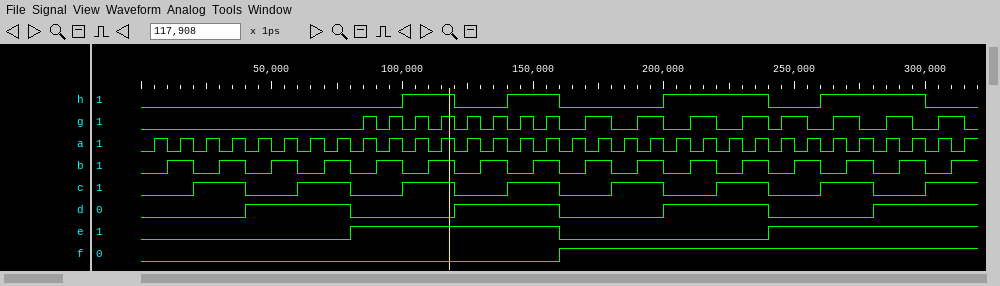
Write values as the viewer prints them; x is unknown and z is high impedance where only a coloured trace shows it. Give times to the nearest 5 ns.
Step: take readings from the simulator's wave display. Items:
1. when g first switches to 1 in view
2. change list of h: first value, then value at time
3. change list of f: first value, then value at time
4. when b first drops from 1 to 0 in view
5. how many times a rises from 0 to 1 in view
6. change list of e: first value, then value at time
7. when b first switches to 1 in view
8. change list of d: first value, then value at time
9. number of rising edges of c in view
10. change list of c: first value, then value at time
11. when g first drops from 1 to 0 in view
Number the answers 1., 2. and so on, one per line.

1. 85 ns
2. 0, 1 at 100 ns, 0 at 120 ns, 1 at 140 ns, 0 at 160 ns, 1 at 200 ns, 0 at 240 ns, 1 at 260 ns, 0 at 300 ns
3. 0, 1 at 160 ns
4. 20 ns
5. 32
6. 0, 1 at 80 ns, 0 at 160 ns, 1 at 240 ns
7. 10 ns
8. 0, 1 at 40 ns, 0 at 80 ns, 1 at 120 ns, 0 at 160 ns, 1 at 200 ns, 0 at 240 ns, 1 at 280 ns
9. 8
10. 0, 1 at 20 ns, 0 at 40 ns, 1 at 60 ns, 0 at 80 ns, 1 at 100 ns, 0 at 120 ns, 1 at 140 ns, 0 at 160 ns, 1 at 180 ns, 0 at 200 ns, 1 at 220 ns, 0 at 240 ns, 1 at 260 ns, 0 at 280 ns, 1 at 300 ns
11. 90 ns
